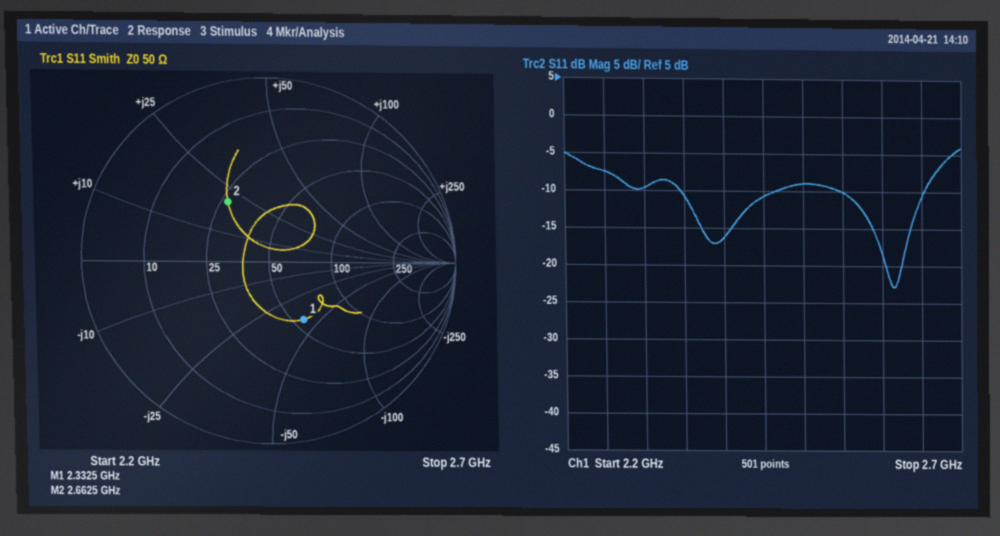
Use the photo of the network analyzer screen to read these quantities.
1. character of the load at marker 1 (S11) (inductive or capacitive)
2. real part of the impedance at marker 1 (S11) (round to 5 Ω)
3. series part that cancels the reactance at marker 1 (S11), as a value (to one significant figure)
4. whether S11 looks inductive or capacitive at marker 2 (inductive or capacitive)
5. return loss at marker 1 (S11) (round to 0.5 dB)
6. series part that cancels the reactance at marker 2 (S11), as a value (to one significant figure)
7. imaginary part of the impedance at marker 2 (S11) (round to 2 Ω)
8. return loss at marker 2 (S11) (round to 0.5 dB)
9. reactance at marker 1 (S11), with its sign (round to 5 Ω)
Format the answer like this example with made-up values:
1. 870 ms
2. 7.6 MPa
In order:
1. capacitive
2. 55 Ω
3. 3 nH
4. inductive
5. 9.0 dB
6. 3 pF
7. +20 Ω
8. 8.0 dB
9. -40 Ω
